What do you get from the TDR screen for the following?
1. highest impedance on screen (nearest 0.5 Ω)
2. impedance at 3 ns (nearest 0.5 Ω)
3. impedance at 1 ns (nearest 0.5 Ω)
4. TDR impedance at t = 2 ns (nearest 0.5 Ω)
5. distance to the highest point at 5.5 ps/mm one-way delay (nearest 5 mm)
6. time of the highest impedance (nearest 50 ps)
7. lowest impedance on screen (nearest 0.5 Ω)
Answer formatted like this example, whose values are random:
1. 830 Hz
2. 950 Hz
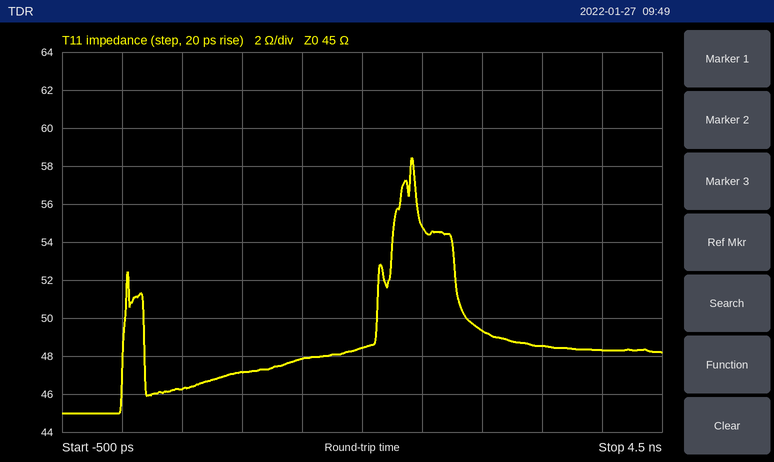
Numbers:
1. 58.5 Ω
2. 49.5 Ω
3. 47.0 Ω
4. 48.5 Ω
5. 220 mm
6. 2.40 ns
7. 45.0 Ω
